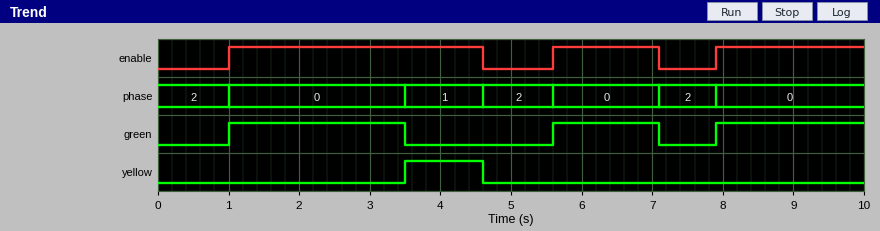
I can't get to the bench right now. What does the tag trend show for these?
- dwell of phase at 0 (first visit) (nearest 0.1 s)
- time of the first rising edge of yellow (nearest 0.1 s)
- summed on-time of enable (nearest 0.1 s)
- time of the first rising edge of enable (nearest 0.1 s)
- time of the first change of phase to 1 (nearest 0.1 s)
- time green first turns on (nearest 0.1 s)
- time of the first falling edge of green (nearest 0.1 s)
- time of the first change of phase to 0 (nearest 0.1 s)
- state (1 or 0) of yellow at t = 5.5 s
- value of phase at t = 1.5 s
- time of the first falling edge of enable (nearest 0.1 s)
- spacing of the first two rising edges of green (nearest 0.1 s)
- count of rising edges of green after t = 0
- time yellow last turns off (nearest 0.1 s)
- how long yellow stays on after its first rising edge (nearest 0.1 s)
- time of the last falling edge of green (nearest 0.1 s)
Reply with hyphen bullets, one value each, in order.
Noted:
- 2.5 s
- 3.5 s
- 7.2 s
- 1.0 s
- 3.5 s
- 1.0 s
- 3.5 s
- 1.0 s
- 0
- 0
- 4.6 s
- 4.6 s
- 3
- 4.6 s
- 1.1 s
- 7.1 s
